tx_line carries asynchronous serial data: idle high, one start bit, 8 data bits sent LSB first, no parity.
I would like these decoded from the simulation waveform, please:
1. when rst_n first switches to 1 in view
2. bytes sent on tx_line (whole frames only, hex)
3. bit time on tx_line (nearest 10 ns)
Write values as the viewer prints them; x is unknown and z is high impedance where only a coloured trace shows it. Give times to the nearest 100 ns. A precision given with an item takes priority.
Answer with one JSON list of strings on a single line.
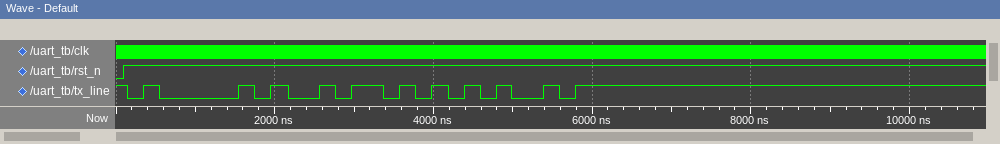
["100 ns", "41, 5A, A5", "200 ns"]
